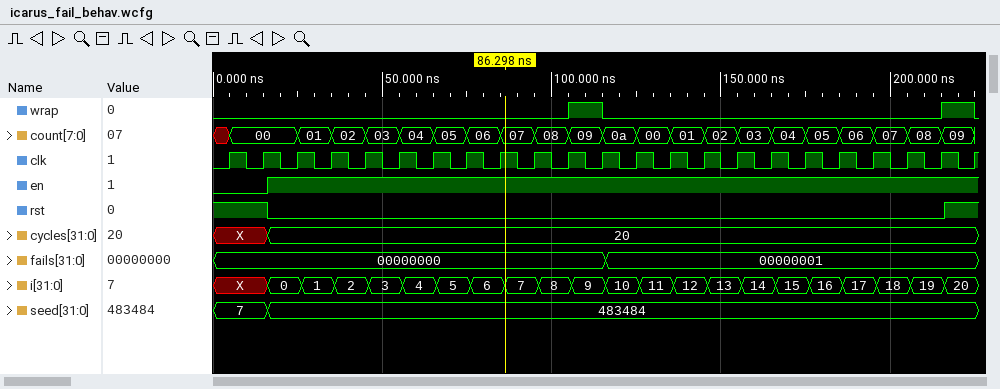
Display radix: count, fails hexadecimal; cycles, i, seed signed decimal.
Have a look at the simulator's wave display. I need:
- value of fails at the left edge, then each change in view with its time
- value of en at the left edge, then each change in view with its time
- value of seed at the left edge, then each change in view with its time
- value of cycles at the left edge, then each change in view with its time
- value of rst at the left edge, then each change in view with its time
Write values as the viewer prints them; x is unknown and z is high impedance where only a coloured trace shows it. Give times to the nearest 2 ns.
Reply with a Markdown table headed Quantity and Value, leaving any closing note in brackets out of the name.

| Quantity | Value |
|---|---|
| value of fails at the left edge, then each change in view with its time | 00000000, 00000001 at 116 ns |
| value of en at the left edge, then each change in view with its time | 0, 1 at 16 ns |
| value of seed at the left edge, then each change in view with its time | 7, 483484 at 16 ns |
| value of cycles at the left edge, then each change in view with its time | X, 20 at 16 ns |
| value of rst at the left edge, then each change in view with its time | 1, 0 at 16 ns, 1 at 216 ns |
